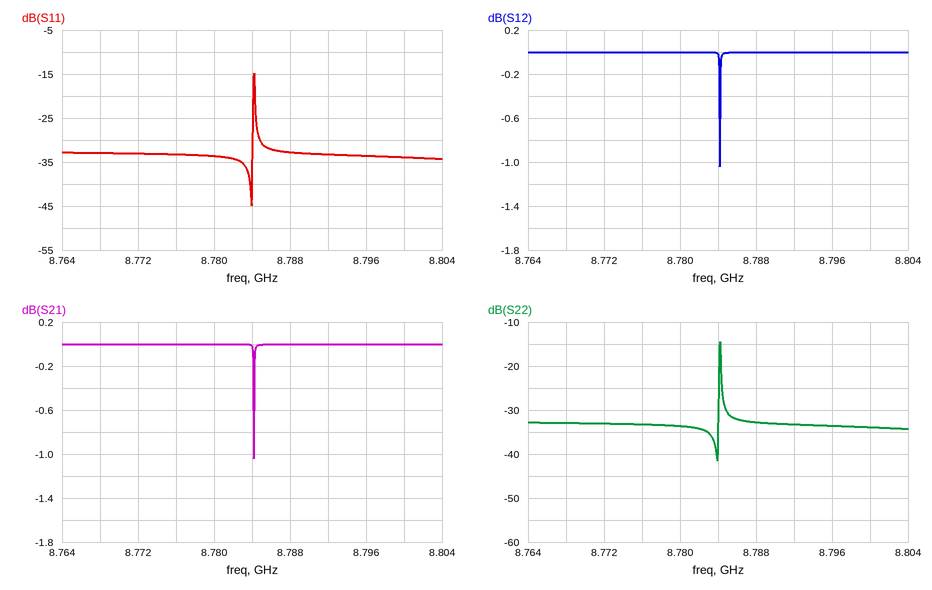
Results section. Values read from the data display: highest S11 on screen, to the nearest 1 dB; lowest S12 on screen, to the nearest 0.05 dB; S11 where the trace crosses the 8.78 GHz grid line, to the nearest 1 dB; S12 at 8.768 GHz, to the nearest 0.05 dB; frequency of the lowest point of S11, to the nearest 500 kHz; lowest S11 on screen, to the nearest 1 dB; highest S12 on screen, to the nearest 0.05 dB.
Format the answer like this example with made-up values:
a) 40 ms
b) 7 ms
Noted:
a) -15 dB
b) -1.05 dB
c) -34 dB
d) 0.00 dB
e) 8.7840 GHz
f) -45 dB
g) 0.00 dB
